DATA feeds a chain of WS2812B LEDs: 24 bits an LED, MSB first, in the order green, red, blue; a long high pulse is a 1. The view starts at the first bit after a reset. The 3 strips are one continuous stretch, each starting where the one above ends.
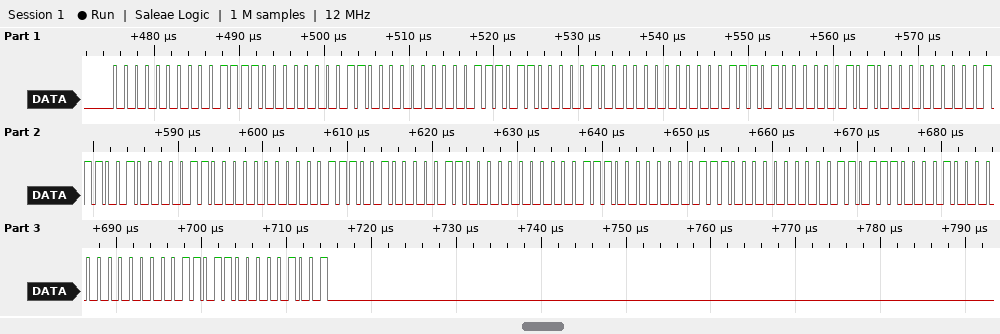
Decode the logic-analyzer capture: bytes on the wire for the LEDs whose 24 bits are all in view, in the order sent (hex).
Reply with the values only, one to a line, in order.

00 3C 03 00 3B 04 00 3A 05 00 39 06 00 39 06 00 38 07 00 37 08 00 36 09
